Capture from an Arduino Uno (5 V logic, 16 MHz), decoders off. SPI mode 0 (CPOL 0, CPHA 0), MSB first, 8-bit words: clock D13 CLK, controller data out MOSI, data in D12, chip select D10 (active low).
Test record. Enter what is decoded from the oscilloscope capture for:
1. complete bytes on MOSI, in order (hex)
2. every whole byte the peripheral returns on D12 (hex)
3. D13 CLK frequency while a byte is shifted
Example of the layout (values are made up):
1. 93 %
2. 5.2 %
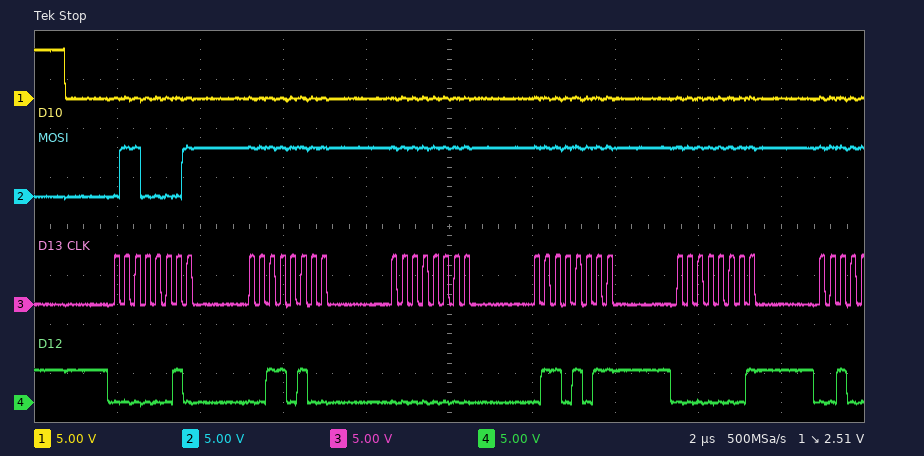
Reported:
1. 61 FF FF FF FF
2. 02 34 00 6B 01
3. 4 MHz
